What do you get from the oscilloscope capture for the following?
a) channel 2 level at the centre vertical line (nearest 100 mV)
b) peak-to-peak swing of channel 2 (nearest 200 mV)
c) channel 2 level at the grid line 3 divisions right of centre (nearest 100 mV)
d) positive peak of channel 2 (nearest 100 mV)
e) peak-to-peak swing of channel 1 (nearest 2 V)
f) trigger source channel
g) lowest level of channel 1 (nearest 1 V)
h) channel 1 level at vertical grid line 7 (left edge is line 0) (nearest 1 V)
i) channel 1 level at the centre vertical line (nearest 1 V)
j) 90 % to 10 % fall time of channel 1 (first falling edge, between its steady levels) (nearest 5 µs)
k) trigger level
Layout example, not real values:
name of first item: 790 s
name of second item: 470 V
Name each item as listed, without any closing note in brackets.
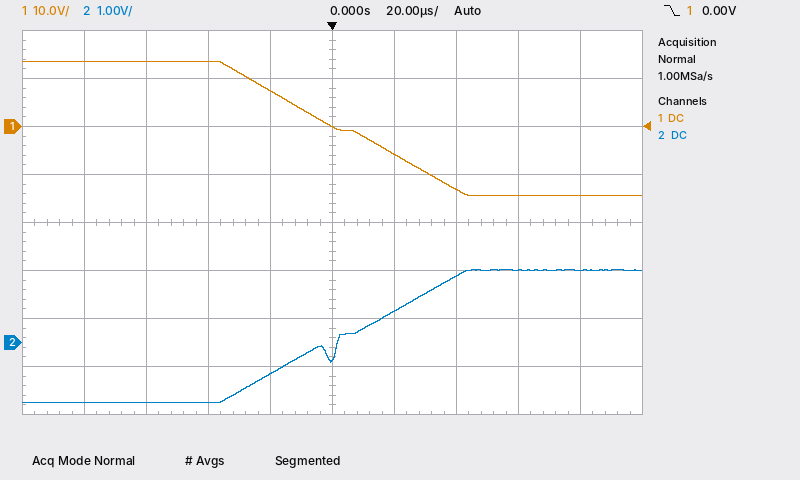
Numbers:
channel 2 level at the centre vertical line: -300 mV
peak-to-peak swing of channel 2: 2.8 V
channel 2 level at the grid line 3 divisions right of centre: 1.5 V
positive peak of channel 2: 1.5 V
peak-to-peak swing of channel 1: 28 V
trigger source channel: channel 1
lowest level of channel 1: -14 V
channel 1 level at vertical grid line 7 (left edge is line 0): -13 V
channel 1 level at the centre vertical line: 0 V
90 % to 10 % fall time of channel 1 (first falling edge, between its steady levels): 65 µs
trigger level: 0.00 V
